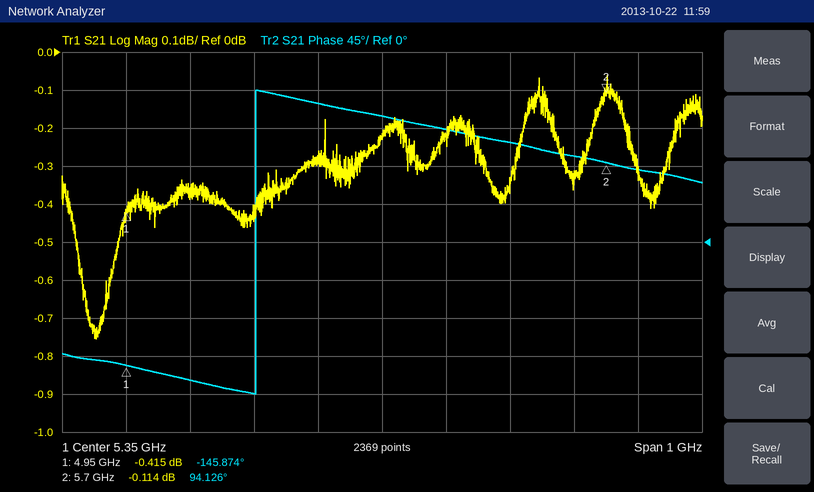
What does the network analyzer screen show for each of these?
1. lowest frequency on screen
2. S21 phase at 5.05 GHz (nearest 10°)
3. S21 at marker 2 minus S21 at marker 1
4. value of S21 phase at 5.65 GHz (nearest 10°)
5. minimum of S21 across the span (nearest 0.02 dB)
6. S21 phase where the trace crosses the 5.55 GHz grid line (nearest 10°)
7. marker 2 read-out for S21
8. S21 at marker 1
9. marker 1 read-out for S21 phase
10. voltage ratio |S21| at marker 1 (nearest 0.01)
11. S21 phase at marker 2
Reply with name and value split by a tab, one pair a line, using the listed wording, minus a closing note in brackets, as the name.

lowest frequency on screen	4.85 GHz
S21 phase at 5.05 GHz	-160°
S21 at marker 2 minus S21 at marker 1	0.301 dB
value of S21 phase at 5.65 GHz	100°
minimum of S21 across the span	-0.76 dB
S21 phase where the trace crosses the 5.55 GHz grid line	120°
marker 2 read-out for S21	-0.114 dB
S21 at marker 1	-0.415 dB
marker 1 read-out for S21 phase	-145.874°
voltage ratio |S21| at marker 1	0.95
S21 phase at marker 2	94.126°
